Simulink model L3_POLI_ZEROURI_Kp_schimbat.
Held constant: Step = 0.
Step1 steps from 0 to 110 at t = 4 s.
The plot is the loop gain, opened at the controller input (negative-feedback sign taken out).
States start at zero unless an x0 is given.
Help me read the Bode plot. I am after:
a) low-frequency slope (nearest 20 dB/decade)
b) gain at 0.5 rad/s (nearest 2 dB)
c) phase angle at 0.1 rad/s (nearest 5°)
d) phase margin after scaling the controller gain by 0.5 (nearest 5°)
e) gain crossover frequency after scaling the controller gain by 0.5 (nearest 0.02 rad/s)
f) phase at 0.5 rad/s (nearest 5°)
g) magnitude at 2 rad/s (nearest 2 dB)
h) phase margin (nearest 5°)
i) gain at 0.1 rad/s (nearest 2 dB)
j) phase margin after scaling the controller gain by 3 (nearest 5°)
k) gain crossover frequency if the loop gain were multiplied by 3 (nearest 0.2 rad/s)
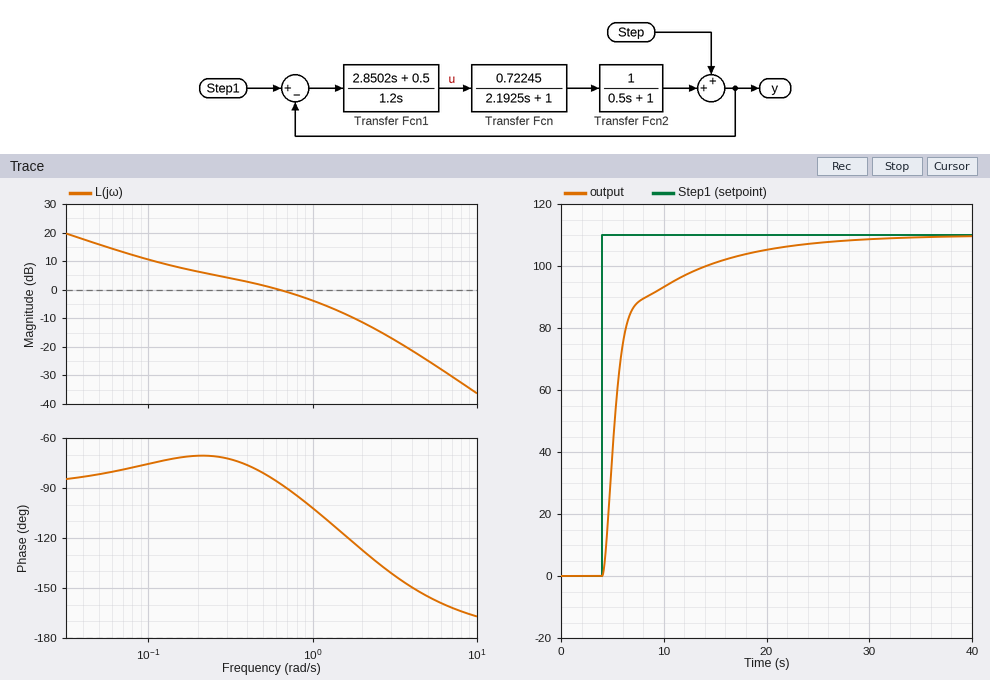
-20 dB/decade
2 dB
-75°
110°
0.22 rad/s
-80°
-12 dB
95°
10 dB
60°
1.8 rad/s
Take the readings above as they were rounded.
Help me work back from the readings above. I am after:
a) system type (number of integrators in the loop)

1
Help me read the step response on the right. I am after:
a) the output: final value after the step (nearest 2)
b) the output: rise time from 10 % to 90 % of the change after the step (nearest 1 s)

110
9 s
